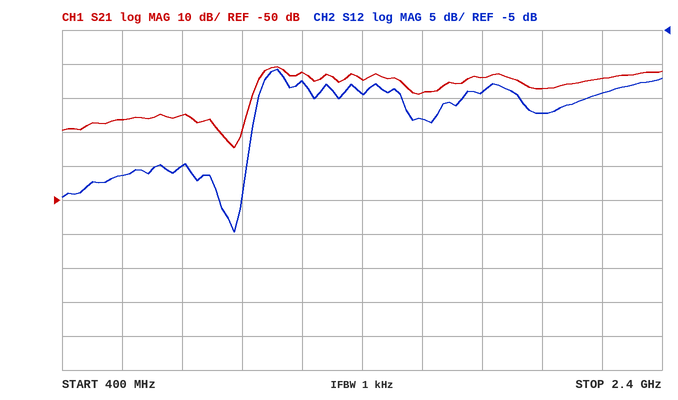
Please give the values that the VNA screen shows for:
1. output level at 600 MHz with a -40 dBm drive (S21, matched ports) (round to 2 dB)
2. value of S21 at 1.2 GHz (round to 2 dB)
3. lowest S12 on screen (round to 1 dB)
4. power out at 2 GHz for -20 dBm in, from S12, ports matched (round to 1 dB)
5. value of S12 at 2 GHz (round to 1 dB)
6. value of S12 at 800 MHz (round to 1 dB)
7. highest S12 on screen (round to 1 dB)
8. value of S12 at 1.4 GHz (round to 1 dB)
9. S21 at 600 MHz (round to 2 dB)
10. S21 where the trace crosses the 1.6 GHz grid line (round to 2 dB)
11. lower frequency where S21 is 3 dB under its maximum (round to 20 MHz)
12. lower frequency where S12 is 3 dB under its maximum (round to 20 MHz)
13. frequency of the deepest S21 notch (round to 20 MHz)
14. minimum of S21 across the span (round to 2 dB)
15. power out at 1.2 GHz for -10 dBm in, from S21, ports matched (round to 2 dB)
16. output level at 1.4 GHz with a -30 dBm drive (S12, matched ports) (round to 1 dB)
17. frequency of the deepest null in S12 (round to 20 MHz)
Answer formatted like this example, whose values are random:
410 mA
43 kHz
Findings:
-66 dBm
-12 dB
-35 dB
-37 dBm
-17 dB
-25 dB
-11 dB
-14 dB
-26 dB
-18 dB
1.06 GHz
1.06 GHz
980 MHz
-34 dB
-22 dBm
-44 dBm
980 MHz
